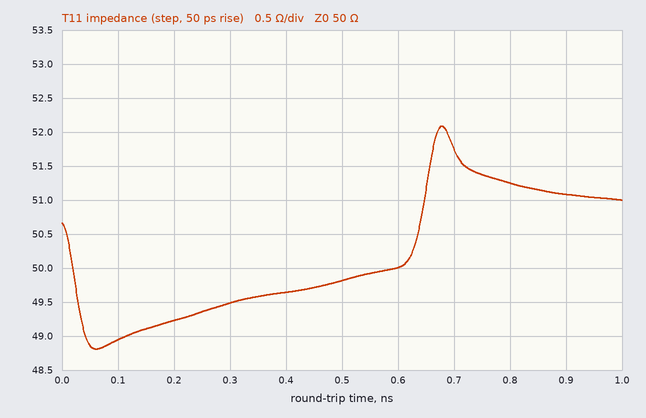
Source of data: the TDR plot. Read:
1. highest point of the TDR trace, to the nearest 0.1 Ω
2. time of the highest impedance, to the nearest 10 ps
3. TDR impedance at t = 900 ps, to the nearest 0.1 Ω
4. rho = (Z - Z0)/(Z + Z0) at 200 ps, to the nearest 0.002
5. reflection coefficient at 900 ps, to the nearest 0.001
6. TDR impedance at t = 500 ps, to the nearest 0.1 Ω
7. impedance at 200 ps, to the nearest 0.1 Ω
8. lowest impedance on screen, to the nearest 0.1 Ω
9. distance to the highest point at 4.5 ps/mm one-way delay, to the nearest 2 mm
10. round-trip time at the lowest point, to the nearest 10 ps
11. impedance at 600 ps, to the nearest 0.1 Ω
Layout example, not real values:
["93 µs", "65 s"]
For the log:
["52.1 Ω", "680 ps", "51.1 Ω", "-0.008", "+0.011", "49.8 Ω", "49.2 Ω", "48.8 Ω", "76 mm", "60 ps", "50.0 Ω"]
